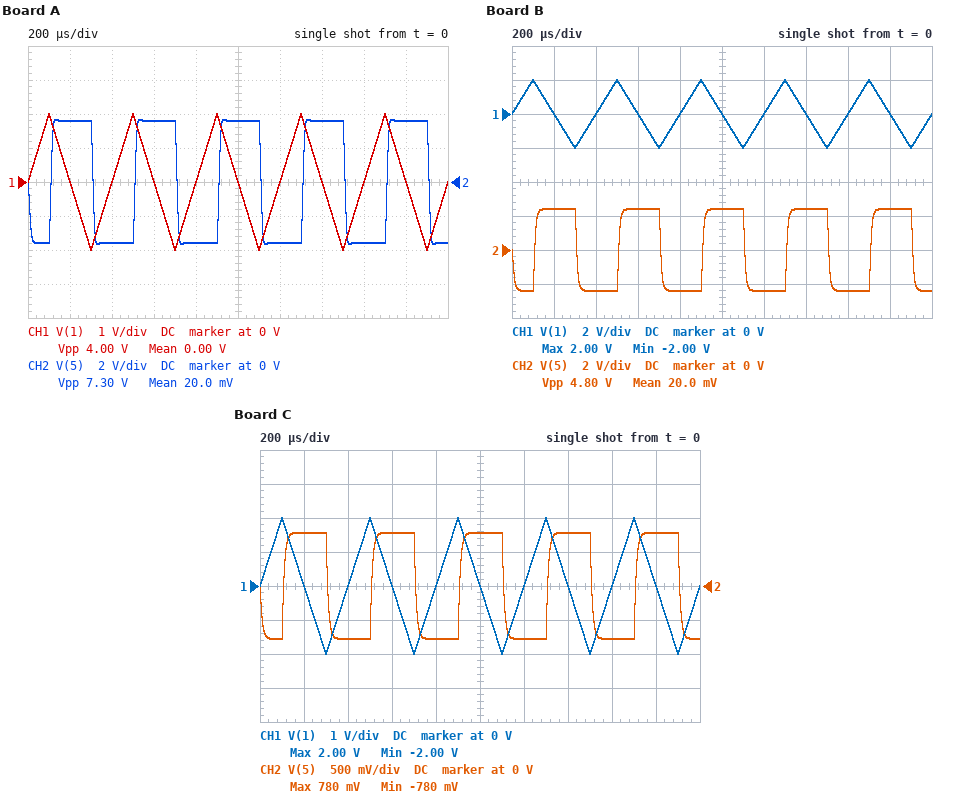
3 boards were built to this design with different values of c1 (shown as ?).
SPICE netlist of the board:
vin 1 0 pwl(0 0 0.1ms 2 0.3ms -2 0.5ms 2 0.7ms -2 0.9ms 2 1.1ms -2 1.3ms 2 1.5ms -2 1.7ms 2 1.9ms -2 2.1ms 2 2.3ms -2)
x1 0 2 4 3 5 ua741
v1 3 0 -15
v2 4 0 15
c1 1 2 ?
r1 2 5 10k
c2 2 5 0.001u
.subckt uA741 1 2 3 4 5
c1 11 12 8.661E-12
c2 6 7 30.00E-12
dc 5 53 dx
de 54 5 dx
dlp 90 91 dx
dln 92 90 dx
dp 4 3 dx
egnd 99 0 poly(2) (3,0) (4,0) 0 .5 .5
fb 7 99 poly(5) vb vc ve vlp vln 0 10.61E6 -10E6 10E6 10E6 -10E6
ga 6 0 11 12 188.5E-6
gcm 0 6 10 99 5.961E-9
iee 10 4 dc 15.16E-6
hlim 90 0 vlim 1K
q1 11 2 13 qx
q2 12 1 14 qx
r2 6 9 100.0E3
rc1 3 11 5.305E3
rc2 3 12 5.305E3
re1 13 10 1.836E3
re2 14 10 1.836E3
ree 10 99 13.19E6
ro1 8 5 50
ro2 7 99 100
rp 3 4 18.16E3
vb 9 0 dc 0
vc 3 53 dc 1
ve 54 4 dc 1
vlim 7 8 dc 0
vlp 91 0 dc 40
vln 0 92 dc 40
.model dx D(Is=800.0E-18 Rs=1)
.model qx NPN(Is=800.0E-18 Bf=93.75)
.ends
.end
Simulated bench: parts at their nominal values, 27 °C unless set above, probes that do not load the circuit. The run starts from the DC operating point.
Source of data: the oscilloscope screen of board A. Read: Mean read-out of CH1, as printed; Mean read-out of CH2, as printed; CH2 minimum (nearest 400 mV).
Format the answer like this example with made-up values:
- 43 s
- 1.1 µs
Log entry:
- 0.00 V
- 20.0 mV
- -3.6 V
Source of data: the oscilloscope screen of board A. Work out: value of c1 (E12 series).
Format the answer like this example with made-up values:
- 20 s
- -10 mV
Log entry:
- 18 nF
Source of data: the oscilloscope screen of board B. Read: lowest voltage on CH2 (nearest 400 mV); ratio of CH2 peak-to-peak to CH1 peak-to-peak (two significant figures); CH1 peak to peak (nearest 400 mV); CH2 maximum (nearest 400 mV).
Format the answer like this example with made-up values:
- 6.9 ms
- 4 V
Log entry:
- -2.4 V
- 1.2
- 4.0 V
- 2.4 V
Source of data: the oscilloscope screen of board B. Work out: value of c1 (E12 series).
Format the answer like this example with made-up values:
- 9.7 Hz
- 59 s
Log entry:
- 12 nF
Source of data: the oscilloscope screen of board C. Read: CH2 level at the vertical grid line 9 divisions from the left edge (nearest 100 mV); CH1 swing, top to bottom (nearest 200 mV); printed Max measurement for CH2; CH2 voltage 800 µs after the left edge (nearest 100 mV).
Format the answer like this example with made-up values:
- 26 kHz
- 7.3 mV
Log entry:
- 800 mV
- 4.0 V
- 780 mV
- -800 mV
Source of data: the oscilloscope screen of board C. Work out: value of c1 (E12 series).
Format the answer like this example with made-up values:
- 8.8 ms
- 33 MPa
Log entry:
- 3.9 nF
